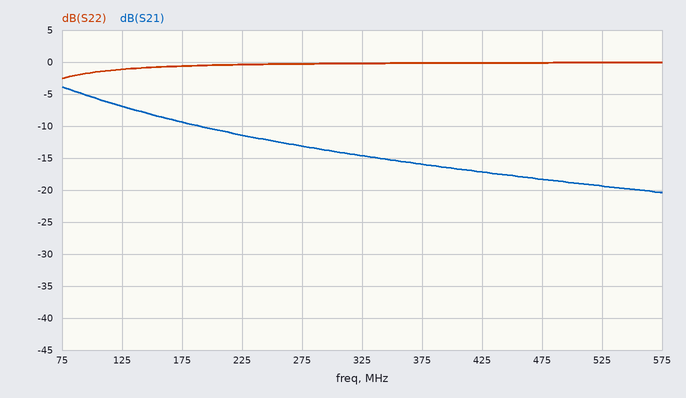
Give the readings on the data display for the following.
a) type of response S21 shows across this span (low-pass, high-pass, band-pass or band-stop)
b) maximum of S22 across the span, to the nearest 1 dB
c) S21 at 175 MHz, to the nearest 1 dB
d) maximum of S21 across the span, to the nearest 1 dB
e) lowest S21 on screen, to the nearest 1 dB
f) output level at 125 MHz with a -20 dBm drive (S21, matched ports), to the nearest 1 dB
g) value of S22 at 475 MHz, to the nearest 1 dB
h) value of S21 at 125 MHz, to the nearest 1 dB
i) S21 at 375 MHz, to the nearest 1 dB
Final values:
low-pass
0 dB
-9 dB
-4 dB
-20 dB
-27 dBm
0 dB
-7 dB
-16 dB
